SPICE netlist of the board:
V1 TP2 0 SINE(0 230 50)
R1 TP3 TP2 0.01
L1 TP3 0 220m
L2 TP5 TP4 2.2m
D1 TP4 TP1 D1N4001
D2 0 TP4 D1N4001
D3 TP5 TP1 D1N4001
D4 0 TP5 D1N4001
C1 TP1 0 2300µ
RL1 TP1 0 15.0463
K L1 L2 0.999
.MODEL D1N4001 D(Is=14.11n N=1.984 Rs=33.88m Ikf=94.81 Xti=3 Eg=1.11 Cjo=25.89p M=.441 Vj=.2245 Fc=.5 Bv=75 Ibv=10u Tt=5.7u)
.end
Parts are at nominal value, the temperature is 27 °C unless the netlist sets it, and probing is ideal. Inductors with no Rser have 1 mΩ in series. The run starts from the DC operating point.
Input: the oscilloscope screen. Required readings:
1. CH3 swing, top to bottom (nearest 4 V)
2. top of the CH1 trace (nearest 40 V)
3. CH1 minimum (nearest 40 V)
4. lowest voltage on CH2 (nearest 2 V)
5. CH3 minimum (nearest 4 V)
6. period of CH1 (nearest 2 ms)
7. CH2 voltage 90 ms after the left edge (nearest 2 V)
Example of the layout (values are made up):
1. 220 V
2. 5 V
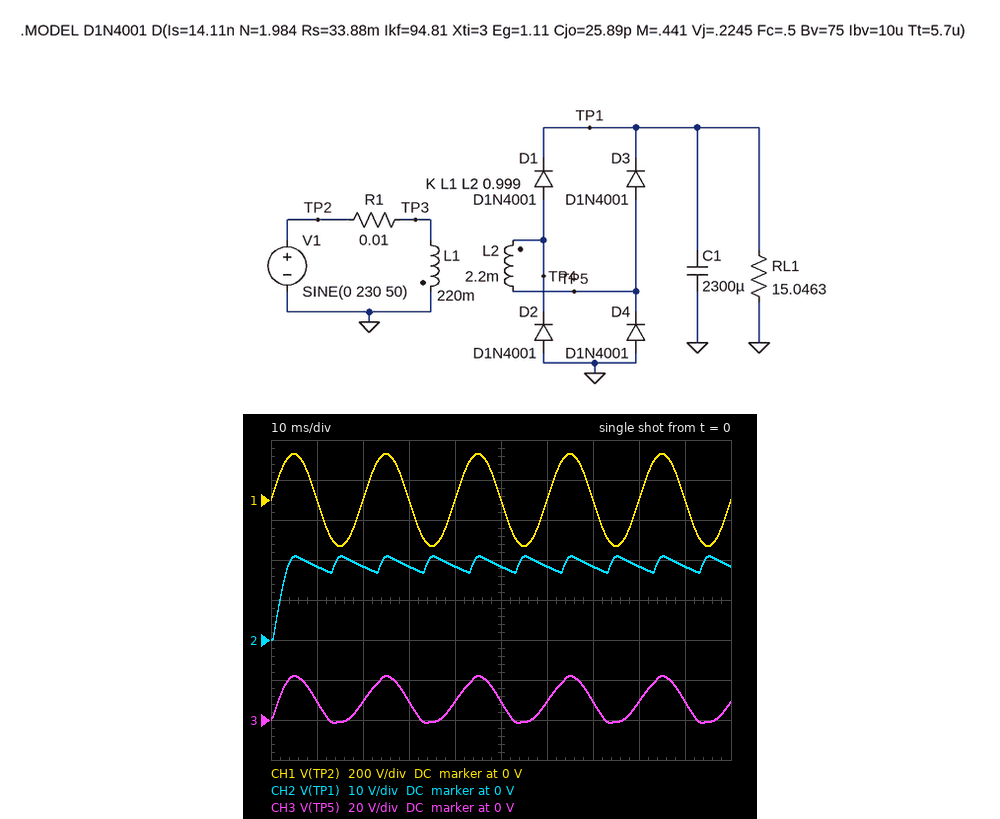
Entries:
1. 24 V
2. 240 V
3. -240 V
4. 0 V
5. 0 V
6. 20 ms
7. 18 V
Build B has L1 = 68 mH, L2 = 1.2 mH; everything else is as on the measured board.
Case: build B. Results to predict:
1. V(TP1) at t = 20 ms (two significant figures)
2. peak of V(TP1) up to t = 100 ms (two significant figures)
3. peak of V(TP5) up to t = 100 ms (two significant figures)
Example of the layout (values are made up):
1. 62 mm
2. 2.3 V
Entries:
1. 25 V
2. 28 V
3. 29 V
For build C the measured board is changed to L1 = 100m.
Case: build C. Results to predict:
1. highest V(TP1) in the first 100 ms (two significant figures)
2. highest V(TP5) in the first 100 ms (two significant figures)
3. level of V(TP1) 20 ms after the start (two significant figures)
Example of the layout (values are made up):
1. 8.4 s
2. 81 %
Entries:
1. 32 V
2. 33 V
3. 28 V
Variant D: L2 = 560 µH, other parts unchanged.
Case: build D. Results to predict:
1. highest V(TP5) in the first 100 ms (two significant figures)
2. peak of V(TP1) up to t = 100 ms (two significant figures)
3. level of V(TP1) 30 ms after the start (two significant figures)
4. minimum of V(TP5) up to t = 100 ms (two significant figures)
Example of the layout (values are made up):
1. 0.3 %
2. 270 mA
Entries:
1. 11 V
2. 9.7 V
3. 8.5 V
4. -1.1 V
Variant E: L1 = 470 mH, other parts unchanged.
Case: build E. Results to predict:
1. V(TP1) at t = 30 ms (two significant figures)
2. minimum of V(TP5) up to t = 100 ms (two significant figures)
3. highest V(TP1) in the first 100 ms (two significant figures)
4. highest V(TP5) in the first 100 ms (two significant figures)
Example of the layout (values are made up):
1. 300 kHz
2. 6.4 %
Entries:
1. 12 V
2. -1.2 V
3. 14 V
4. 15 V
